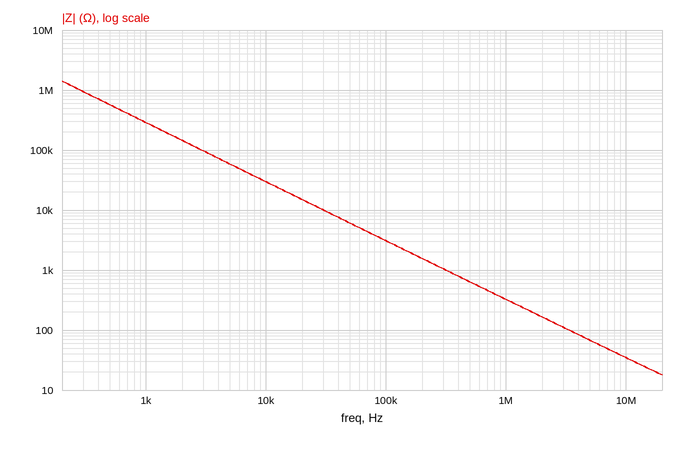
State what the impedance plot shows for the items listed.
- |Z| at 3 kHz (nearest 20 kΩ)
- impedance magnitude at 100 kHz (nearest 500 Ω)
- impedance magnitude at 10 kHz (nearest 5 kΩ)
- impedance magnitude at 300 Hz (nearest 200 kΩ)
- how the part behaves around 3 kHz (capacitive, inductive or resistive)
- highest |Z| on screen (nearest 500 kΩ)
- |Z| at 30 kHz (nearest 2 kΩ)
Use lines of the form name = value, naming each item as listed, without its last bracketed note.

|Z| at 3 kHz = 100 kΩ
impedance magnitude at 100 kHz = 3.0 kΩ
impedance magnitude at 10 kHz = 30 kΩ
impedance magnitude at 300 Hz = 1.0 MΩ
how the part behaves around 3 kHz = capacitive
highest |Z| on screen = 1.5 MΩ
|Z| at 30 kHz = 10 kΩ
